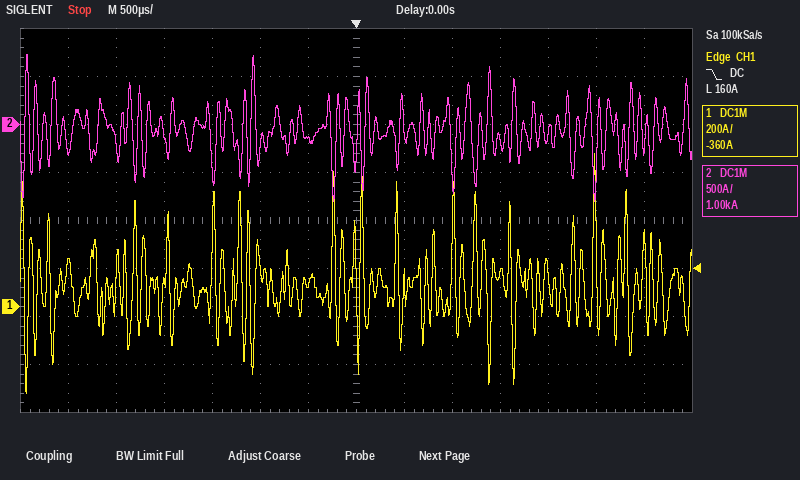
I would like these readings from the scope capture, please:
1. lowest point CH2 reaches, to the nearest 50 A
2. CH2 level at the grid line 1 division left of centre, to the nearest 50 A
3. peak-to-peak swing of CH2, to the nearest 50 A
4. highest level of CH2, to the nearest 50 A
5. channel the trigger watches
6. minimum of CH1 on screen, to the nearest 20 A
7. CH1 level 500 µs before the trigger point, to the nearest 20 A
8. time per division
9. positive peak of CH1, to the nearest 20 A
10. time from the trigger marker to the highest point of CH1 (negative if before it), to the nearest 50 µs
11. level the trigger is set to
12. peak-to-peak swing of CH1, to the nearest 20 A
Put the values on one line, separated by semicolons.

-800 A; -150 A; 1.55 kA; 750 A; CH1; -360 A; 100 A; 500 µs; 640 A; +2.50 ms; 160 A; 1.00 kA
